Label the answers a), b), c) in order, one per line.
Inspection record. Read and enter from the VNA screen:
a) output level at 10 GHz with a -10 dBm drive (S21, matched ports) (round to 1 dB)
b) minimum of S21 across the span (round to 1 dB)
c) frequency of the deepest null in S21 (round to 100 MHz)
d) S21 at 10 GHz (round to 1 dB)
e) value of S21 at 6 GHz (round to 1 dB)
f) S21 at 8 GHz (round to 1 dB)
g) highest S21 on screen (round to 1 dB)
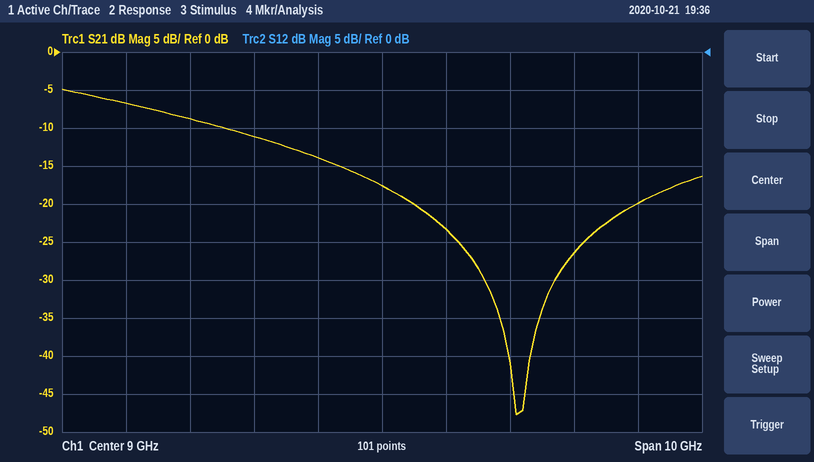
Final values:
a) -33 dBm
b) -48 dB
c) 11.1 GHz
d) -23 dB
e) -9 dB
f) -14 dB
g) -5 dB
